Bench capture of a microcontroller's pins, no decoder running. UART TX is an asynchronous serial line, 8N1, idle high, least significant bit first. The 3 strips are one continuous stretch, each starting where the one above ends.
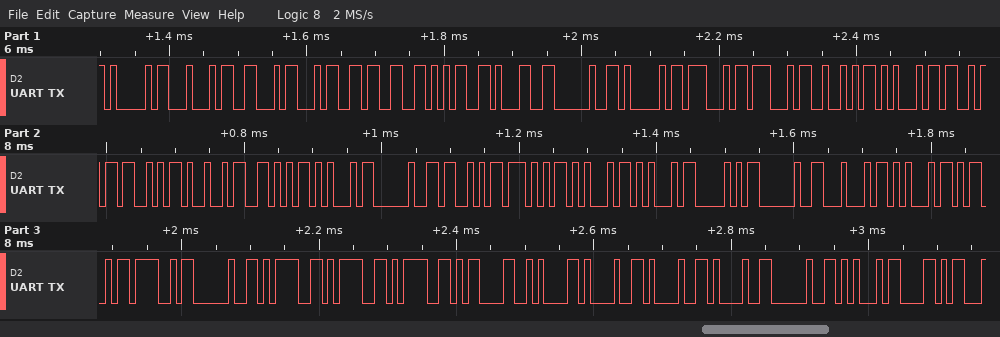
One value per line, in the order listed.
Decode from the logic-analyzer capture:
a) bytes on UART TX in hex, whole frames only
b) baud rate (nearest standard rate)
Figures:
0x41 0x44 0x46 0x34 0x33 0x35 0x31 0x20 0x41 0x47 0x47 0x52 0x45 0x53 0x53 0x49 0x56 0x45 0x20 0x53 0x57 0x45 0x45 0x50 0x20 0x44 0x45 0x4D 0x4F 0x20 0x3D 0x3D 0x3D 0x0D 0x0A 0x21 0x21 0x21 0x20 0x45 0x58
115200 baud
